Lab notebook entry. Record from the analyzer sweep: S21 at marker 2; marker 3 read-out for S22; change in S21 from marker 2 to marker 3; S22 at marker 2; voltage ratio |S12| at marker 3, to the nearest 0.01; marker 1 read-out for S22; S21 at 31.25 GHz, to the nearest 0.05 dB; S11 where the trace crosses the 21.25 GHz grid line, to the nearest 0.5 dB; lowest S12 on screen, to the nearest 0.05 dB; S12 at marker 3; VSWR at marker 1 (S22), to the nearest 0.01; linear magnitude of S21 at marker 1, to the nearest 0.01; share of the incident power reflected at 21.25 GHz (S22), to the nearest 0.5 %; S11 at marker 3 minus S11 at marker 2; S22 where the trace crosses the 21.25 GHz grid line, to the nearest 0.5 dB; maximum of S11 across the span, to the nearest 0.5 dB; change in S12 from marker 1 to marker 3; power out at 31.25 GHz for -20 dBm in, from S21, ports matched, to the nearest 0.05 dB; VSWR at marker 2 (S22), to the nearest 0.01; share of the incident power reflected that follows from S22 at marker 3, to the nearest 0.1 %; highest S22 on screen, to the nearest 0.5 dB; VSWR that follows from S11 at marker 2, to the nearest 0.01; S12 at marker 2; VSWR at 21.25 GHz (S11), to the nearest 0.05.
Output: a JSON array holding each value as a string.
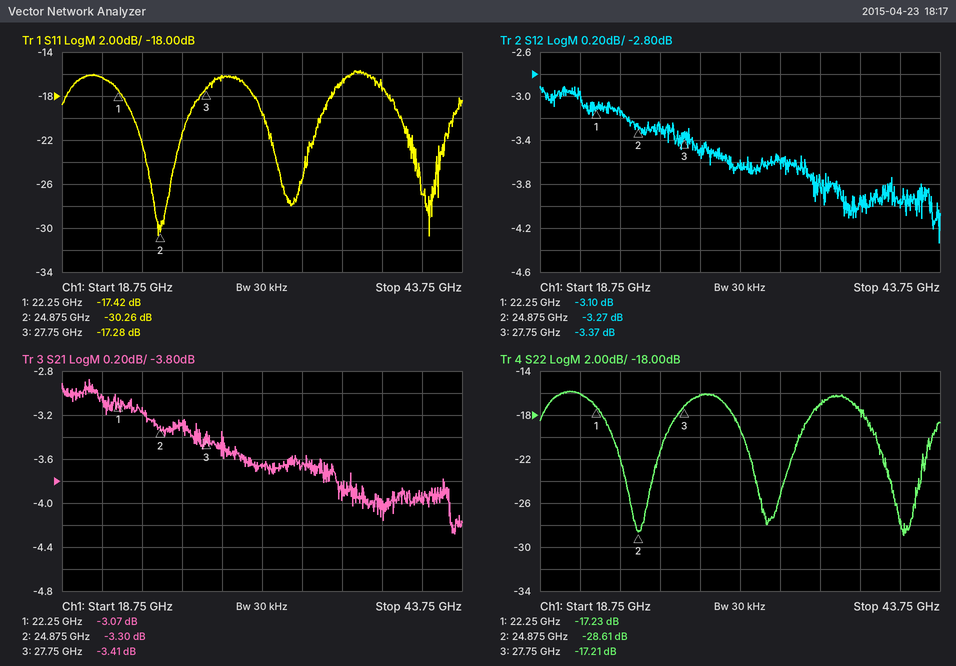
["-3.30 dB", "-17.21 dB", "-0.11 dB", "-28.61 dB", "0.68", "-17.23 dB", "-3.65 dB", "-16.5 dB", "-4.35 dB", "-3.37 dB", "1.32", "0.70", "2.5 %", "12.98 dB", "-16.0 dB", "-15.5 dB", "-0.27 dB", "-23.65 dBm", "1.08", "1.9 %", "-16.0 dB", "1.06", "-3.27 dB", "1.35"]
